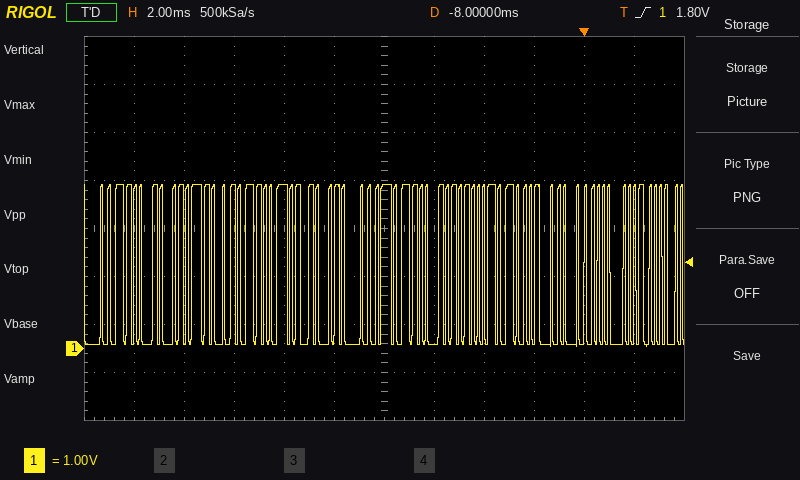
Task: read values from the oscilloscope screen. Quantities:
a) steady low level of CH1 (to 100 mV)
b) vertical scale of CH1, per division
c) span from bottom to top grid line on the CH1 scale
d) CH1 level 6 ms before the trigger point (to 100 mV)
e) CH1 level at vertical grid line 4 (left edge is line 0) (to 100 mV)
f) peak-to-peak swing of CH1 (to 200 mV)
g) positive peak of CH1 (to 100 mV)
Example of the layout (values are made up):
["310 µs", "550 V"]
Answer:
["100 mV", "1 V", "8 V", "100 mV", "3.4 V", "3.4 V", "3.4 V"]
